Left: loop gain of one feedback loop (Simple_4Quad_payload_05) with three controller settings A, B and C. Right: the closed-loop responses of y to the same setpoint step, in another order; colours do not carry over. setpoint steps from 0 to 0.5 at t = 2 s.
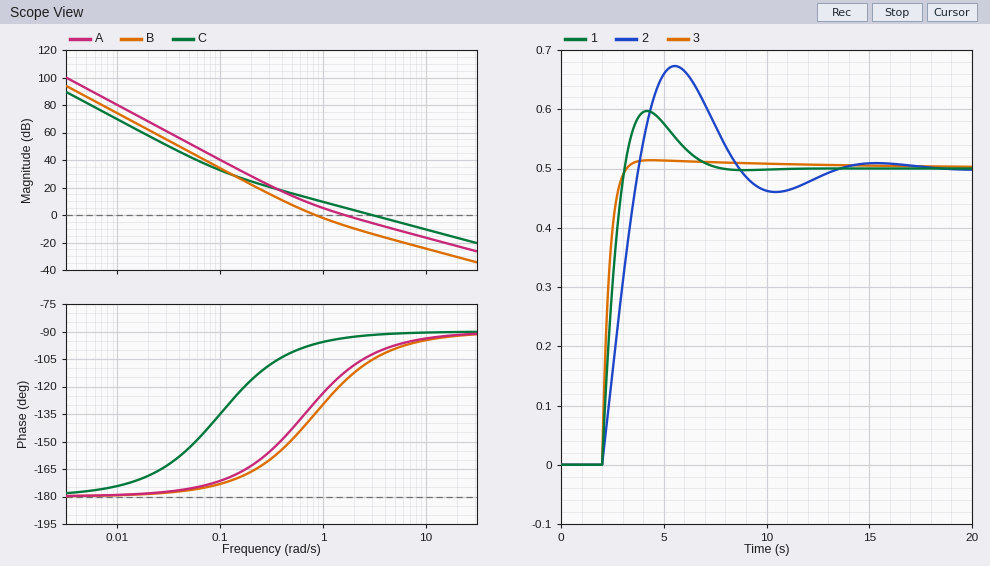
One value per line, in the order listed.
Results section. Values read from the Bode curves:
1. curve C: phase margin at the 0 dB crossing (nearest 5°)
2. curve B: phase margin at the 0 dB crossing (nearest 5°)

90°
45°
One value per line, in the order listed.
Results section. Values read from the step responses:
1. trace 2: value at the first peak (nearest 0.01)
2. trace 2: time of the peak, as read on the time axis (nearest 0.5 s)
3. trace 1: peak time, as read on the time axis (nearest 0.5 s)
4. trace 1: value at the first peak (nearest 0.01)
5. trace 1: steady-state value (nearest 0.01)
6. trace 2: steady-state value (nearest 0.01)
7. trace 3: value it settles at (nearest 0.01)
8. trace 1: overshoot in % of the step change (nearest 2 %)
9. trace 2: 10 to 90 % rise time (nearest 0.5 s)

0.67
5.5 s
4.0 s
0.60
0.50
0.50
0.50
20 %
1.5 s
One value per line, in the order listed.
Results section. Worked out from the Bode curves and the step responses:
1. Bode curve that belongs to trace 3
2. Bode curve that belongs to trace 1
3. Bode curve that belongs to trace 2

C
A
B
